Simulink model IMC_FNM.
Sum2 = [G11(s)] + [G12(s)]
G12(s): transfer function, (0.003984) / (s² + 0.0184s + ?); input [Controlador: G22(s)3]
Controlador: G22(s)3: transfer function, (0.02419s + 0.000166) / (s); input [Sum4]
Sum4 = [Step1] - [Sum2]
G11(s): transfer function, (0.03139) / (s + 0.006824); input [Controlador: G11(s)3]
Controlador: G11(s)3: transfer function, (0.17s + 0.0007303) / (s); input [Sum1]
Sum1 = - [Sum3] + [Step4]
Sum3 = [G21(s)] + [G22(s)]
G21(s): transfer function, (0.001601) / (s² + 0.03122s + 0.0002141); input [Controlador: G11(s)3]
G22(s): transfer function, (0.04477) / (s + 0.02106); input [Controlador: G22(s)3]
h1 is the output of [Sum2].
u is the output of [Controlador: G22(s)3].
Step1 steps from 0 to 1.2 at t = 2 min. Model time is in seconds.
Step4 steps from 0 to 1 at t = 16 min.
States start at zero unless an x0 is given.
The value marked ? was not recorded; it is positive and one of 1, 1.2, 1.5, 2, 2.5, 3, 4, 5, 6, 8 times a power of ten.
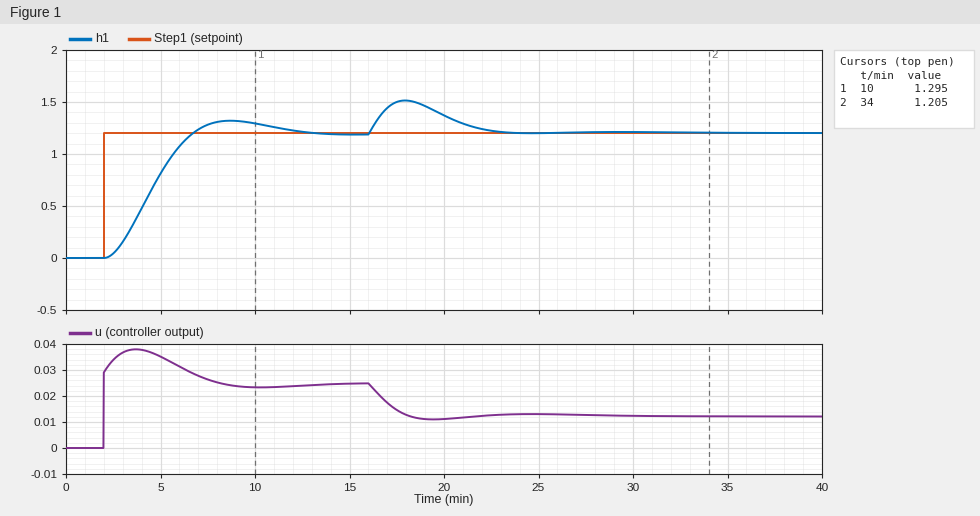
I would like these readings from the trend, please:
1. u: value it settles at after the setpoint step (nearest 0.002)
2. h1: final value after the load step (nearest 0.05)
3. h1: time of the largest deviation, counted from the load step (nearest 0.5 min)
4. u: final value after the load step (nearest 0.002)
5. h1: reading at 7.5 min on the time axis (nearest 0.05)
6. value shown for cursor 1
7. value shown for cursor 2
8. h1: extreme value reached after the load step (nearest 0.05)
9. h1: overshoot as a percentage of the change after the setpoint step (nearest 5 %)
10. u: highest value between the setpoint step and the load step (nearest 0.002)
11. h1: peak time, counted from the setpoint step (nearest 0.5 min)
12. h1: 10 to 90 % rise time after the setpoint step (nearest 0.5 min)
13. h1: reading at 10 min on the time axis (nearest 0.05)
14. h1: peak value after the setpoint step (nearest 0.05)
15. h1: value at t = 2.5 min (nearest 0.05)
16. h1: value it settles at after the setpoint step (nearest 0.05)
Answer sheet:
0.024
1.20
2.0 min
0.012
1.30
1.295
1.205
1.50
10 %
0.038
6.5 min
3.0 min
1.30
1.30
0.05
1.20
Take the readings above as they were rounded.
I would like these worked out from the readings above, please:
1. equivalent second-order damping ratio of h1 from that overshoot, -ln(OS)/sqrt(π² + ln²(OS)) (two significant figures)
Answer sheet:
0.59
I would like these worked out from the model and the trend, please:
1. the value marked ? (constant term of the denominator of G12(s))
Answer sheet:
8e-05
